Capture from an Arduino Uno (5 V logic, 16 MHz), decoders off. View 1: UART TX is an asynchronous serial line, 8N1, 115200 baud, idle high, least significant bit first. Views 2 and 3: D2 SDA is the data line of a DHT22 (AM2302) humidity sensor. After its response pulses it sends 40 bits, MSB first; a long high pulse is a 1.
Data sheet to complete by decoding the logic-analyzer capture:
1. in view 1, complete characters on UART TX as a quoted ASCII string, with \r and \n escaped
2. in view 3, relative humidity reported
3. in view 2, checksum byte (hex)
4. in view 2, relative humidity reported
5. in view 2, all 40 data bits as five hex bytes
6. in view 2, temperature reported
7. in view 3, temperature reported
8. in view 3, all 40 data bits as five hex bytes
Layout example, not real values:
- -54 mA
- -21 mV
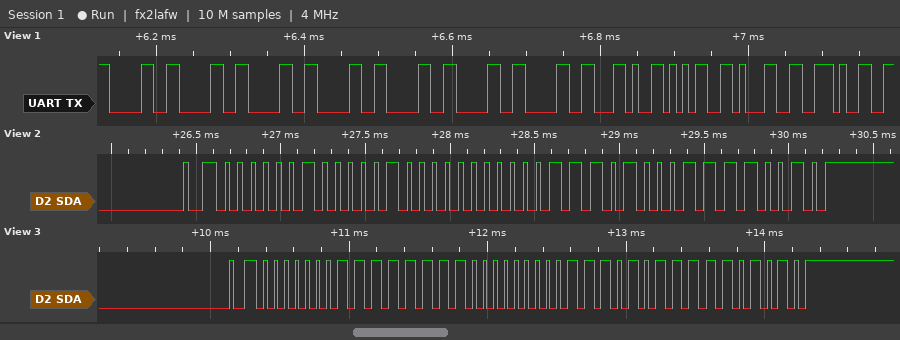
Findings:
- "0000000,51."
- 51.0 %
- 0xF2
- 52.0 %
- 02 08 00 E8 F2
- 23.2 °C
- 23.5 °C
- 01 FE 00 EB EA
